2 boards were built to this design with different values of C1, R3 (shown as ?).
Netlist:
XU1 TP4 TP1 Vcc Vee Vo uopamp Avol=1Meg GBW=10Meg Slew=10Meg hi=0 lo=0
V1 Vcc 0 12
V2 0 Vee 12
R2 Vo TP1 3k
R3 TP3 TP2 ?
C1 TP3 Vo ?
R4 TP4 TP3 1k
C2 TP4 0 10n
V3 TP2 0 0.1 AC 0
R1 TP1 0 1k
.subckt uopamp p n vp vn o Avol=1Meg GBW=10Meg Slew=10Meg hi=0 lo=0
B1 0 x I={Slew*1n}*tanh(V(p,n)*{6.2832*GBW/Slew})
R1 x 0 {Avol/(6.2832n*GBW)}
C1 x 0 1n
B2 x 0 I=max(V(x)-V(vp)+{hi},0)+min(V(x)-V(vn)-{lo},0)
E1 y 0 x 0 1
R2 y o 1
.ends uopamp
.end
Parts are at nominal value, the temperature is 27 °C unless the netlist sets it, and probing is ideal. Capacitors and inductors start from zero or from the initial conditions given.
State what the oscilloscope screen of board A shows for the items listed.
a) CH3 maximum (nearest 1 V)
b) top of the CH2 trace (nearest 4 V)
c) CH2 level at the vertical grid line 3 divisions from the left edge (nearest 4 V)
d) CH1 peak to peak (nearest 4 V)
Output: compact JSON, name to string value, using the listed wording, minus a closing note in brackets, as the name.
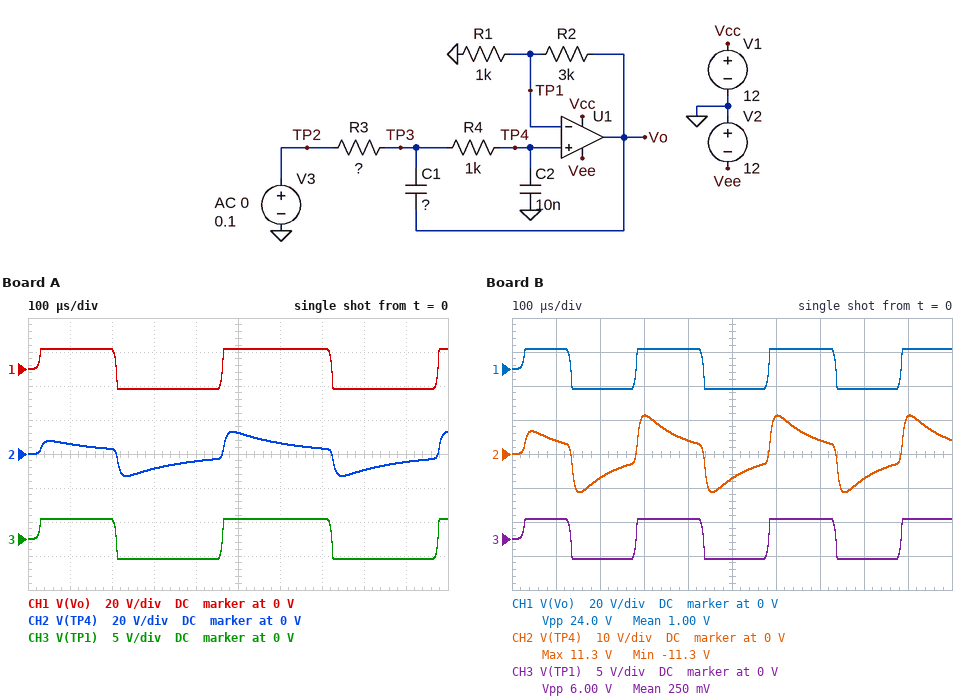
{"CH3 maximum": "3 V", "top of the CH2 trace": "12 V", "CH2 level at the vertical grid line 3 divisions from the left edge": "-8 V", "CH1 peak to peak": "24 V"}
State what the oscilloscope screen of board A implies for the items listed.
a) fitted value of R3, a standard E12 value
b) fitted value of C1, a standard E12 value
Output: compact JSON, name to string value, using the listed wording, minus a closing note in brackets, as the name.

{"fitted value of R3, a standard E12 value": "3.3 kΩ", "fitted value of C1, a standard E12 value": "33 nF"}
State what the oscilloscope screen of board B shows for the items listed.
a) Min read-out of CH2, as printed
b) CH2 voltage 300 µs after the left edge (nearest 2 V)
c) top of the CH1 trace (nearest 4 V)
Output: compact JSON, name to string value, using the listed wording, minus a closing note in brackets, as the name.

{"Min read-out of CH2, as printed": "-11.3 V", "CH2 voltage 300 µs after the left edge": "12 V", "top of the CH1 trace": "12 V"}
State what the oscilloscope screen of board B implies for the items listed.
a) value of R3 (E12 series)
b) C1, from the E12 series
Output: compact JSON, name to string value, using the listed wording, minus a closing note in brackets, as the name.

{"value of R3": "2.2 kΩ", "C1, from the E12 series": "27 nF"}
